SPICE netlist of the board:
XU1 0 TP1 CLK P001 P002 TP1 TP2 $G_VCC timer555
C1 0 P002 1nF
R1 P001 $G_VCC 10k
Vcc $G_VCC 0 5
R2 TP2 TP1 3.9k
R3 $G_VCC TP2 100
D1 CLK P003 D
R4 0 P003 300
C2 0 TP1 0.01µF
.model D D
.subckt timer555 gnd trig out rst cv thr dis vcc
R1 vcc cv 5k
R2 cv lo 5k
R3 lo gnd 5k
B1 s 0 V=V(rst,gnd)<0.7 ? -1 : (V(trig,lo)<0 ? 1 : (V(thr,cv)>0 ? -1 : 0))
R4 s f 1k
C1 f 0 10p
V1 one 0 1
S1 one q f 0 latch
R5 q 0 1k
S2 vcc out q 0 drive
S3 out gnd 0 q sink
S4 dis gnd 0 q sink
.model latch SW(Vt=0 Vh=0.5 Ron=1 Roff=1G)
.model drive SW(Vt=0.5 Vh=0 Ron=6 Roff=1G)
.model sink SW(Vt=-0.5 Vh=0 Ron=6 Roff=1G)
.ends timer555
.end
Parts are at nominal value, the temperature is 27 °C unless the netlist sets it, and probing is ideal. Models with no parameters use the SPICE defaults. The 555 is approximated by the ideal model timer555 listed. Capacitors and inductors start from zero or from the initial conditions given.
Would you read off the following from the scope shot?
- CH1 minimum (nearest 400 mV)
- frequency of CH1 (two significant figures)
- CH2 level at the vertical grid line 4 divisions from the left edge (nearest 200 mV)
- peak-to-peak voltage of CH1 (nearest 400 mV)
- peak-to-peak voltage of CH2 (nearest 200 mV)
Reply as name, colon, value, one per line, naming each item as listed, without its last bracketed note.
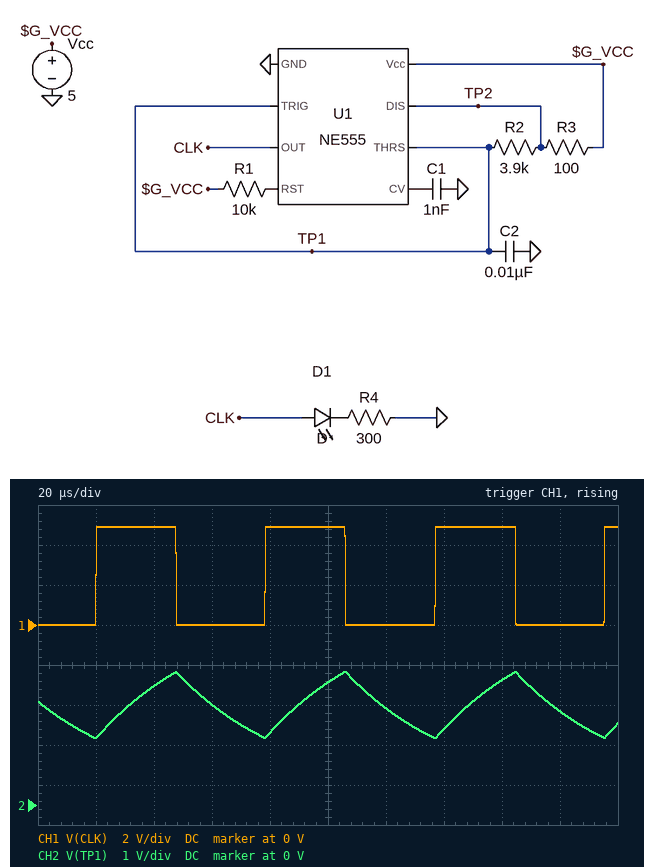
CH1 minimum: 0 V
frequency of CH1: 17 kHz
CH2 level at the vertical grid line 4 divisions from the left edge: 1.8 V
peak-to-peak voltage of CH1: 4.8 V
peak-to-peak voltage of CH2: 1.6 V
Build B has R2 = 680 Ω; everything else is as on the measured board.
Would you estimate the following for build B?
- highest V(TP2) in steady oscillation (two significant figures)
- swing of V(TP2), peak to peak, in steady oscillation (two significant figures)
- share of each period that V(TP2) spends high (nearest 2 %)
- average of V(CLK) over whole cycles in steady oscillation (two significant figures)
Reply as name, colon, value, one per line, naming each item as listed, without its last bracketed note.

highest V(TP2) in steady oscillation: 4.8 V
swing of V(TP2), peak to peak, in steady oscillation: 4.5 V
share of each period that V(TP2) spends high: 50 %
average of V(CLK) over whole cycles in steady oscillation: 2.5 V
